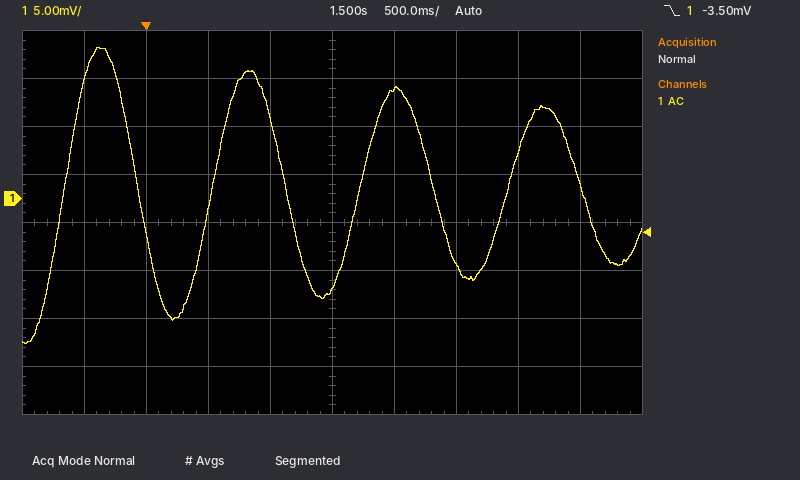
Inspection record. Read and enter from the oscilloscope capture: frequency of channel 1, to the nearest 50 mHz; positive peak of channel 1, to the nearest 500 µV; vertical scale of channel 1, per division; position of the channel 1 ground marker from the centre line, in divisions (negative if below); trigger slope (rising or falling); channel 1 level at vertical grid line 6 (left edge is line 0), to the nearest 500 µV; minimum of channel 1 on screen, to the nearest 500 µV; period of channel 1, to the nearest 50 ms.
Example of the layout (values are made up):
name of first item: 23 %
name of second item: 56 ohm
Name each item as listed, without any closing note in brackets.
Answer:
frequency of channel 1, to the nearest 50 mHz: 850 mHz
positive peak of channel 1, to the nearest 500 µV: 15.5 mV
vertical scale of channel 1, per division: 5 mV
position of the channel 1 ground marker from the centre line, in divisions: +0.5 div
trigger slope: falling
channel 1 level at vertical grid line 6 (left edge is line 0), to the nearest 500 µV: 11.5 mV
minimum of channel 1 on screen, to the nearest 500 µV: -15.0 mV
period of channel 1, to the nearest 50 ms: 1.20 s
